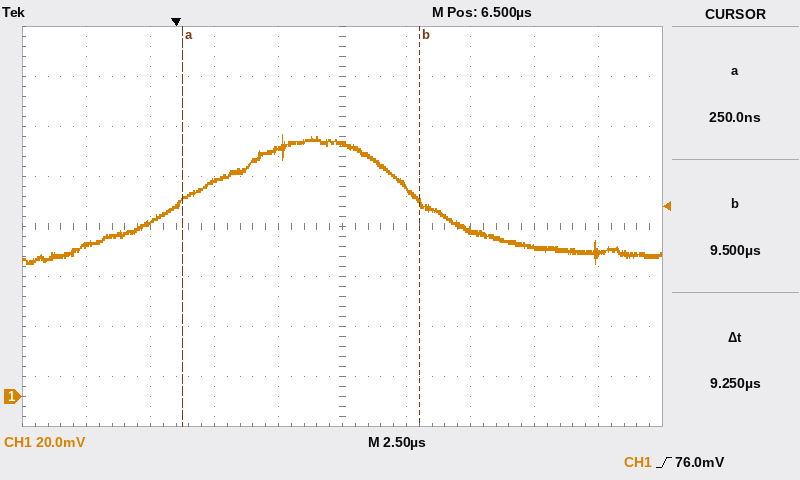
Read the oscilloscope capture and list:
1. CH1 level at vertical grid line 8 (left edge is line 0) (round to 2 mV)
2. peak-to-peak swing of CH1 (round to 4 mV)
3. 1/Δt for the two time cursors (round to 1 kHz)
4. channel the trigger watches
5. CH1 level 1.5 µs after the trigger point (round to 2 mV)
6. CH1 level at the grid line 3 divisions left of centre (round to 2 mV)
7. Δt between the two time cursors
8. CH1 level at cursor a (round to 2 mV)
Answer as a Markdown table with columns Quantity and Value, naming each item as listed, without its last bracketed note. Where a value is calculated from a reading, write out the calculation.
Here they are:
| Quantity | Value |
|---|---|
| CH1 level at vertical grid line 8 (left edge is line 0) | 60 mV |
| peak-to-peak swing of CH1 | 52 mV |
| 1/Δt for the two time cursors | 1 / 9.25 µs ≈ 108 kHz |
| channel the trigger watches | CH1 |
| CH1 level 1.5 µs after the trigger point | 86 mV |
| CH1 level at the grid line 3 divisions left of centre | 70 mV |
| Δt between the two time cursors | 9.25 µs |
| CH1 level at cursor a | 78 mV |
